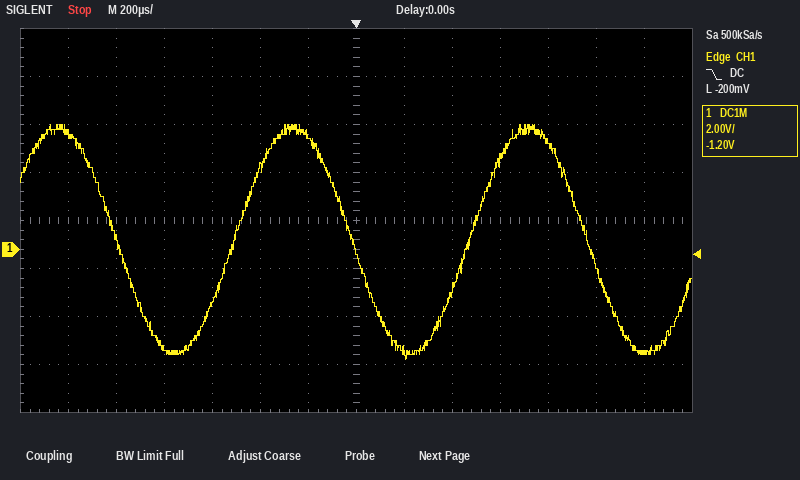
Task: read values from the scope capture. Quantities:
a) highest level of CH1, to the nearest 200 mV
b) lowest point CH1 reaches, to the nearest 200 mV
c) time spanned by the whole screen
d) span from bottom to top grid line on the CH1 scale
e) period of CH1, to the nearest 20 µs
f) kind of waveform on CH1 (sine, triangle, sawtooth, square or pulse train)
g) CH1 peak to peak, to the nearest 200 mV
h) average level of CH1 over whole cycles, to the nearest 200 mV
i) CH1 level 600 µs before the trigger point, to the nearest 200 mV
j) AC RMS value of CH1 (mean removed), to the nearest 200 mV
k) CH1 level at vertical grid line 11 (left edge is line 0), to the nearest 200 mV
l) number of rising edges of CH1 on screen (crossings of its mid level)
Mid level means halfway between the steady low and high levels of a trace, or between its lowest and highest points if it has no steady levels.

5.2 V
-4.6 V
2.8 ms
16 V
980 µs
sine
9.8 V
400 mV
-2.2 V
3.4 V
4.4 V
2
